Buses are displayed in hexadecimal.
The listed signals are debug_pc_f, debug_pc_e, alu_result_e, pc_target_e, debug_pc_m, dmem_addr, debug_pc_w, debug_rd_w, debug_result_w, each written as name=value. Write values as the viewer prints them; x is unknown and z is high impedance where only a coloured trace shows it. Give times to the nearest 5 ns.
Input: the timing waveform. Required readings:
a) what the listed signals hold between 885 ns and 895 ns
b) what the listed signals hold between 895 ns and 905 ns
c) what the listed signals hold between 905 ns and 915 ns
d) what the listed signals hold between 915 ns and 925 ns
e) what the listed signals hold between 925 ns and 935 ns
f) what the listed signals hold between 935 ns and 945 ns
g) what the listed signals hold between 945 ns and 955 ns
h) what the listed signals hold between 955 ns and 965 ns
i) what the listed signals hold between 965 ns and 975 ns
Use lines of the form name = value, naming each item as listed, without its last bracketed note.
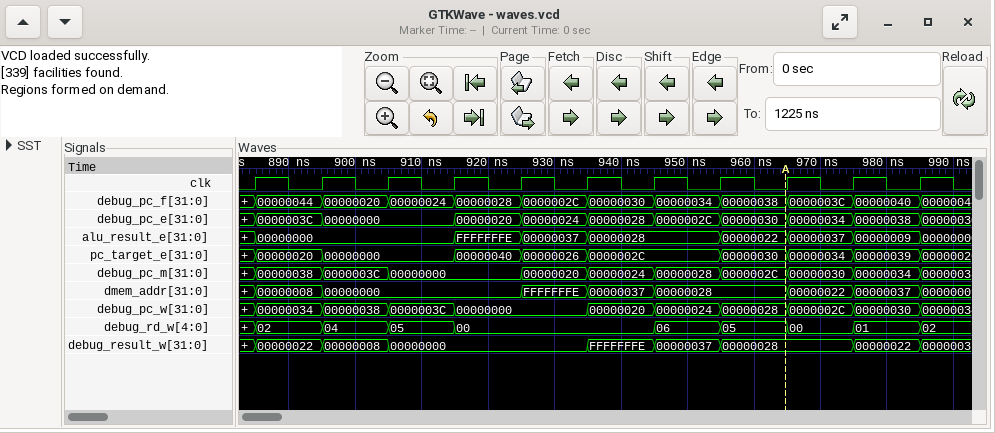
what the listed signals hold between 885 ns and 895 ns = debug_pc_f=00000044, debug_pc_e=0000003C, alu_result_e=00000000, pc_target_e=00000020, debug_pc_m=00000038, dmem_addr=00000008, debug_pc_w=00000034, debug_rd_w=02, debug_result_w=00000022
what the listed signals hold between 895 ns and 905 ns = debug_pc_f=00000020, debug_pc_e=00000000, alu_result_e=00000000, pc_target_e=00000000, debug_pc_m=0000003C, dmem_addr=00000000, debug_pc_w=00000038, debug_rd_w=04, debug_result_w=00000008
what the listed signals hold between 905 ns and 915 ns = debug_pc_f=00000024, debug_pc_e=00000000, alu_result_e=00000000, pc_target_e=00000000, debug_pc_m=00000000, dmem_addr=00000000, debug_pc_w=0000003C, debug_rd_w=05, debug_result_w=00000000
what the listed signals hold between 915 ns and 925 ns = debug_pc_f=00000028, debug_pc_e=00000020, alu_result_e=FFFFFFFE, pc_target_e=00000040, debug_pc_m=00000000, dmem_addr=00000000, debug_pc_w=00000000, debug_rd_w=00, debug_result_w=00000000
what the listed signals hold between 925 ns and 935 ns = debug_pc_f=0000002C, debug_pc_e=00000024, alu_result_e=00000037, pc_target_e=00000026, debug_pc_m=00000020, dmem_addr=FFFFFFFE, debug_pc_w=00000000, debug_rd_w=00, debug_result_w=00000000
what the listed signals hold between 935 ns and 945 ns = debug_pc_f=00000030, debug_pc_e=00000028, alu_result_e=00000028, pc_target_e=0000002C, debug_pc_m=00000024, dmem_addr=00000037, debug_pc_w=00000020, debug_rd_w=00, debug_result_w=FFFFFFFE
what the listed signals hold between 945 ns and 955 ns = debug_pc_f=00000034, debug_pc_e=0000002C, alu_result_e=00000028, pc_target_e=0000002C, debug_pc_m=00000028, dmem_addr=00000028, debug_pc_w=00000024, debug_rd_w=06, debug_result_w=00000037
what the listed signals hold between 955 ns and 965 ns = debug_pc_f=00000038, debug_pc_e=00000030, alu_result_e=00000022, pc_target_e=00000030, debug_pc_m=0000002C, dmem_addr=00000028, debug_pc_w=00000028, debug_rd_w=05, debug_result_w=00000028
what the listed signals hold between 965 ns and 975 ns = debug_pc_f=0000003C, debug_pc_e=00000034, alu_result_e=00000037, pc_target_e=00000034, debug_pc_m=00000030, dmem_addr=00000022, debug_pc_w=0000002C, debug_rd_w=00, debug_result_w=00000028
